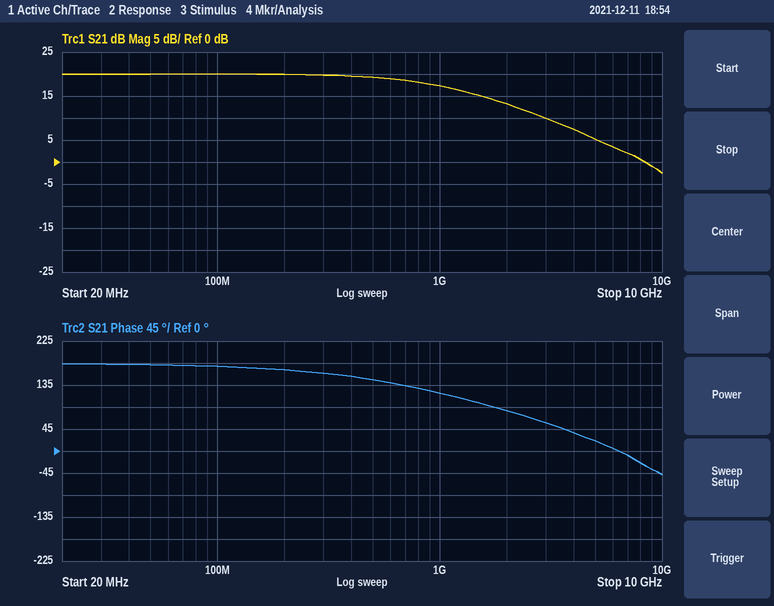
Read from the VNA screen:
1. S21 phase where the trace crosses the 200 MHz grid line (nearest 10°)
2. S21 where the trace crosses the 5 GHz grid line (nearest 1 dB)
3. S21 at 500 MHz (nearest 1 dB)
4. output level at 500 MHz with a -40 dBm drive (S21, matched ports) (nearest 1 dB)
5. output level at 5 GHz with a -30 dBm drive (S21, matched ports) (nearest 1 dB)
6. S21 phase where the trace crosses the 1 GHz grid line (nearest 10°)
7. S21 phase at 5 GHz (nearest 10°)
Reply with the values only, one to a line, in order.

170°
5 dB
19 dB
-21 dBm
-25 dBm
120°
20°
